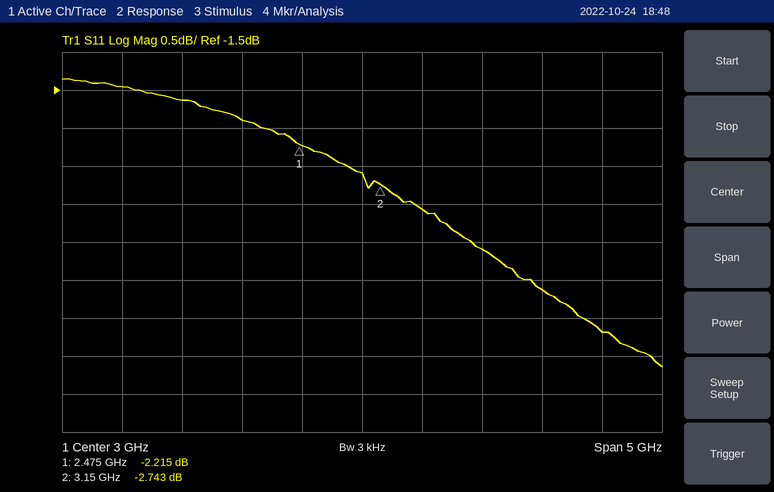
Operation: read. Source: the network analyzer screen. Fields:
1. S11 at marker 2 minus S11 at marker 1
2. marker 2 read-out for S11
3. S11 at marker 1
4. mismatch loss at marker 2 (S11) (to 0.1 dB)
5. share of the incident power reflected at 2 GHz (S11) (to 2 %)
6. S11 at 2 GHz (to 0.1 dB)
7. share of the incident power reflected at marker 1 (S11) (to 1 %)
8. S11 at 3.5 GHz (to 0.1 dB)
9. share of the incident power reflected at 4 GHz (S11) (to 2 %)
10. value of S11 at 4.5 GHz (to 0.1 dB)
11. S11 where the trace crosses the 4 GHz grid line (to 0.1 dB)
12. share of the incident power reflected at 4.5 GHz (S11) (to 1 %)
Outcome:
-0.528 dB
-2.743 dB
-2.215 dB
3.3 dB
64 %
-1.9 dB
60 %
-3.1 dB
44 %
-4.1 dB
-3.6 dB
39 %
